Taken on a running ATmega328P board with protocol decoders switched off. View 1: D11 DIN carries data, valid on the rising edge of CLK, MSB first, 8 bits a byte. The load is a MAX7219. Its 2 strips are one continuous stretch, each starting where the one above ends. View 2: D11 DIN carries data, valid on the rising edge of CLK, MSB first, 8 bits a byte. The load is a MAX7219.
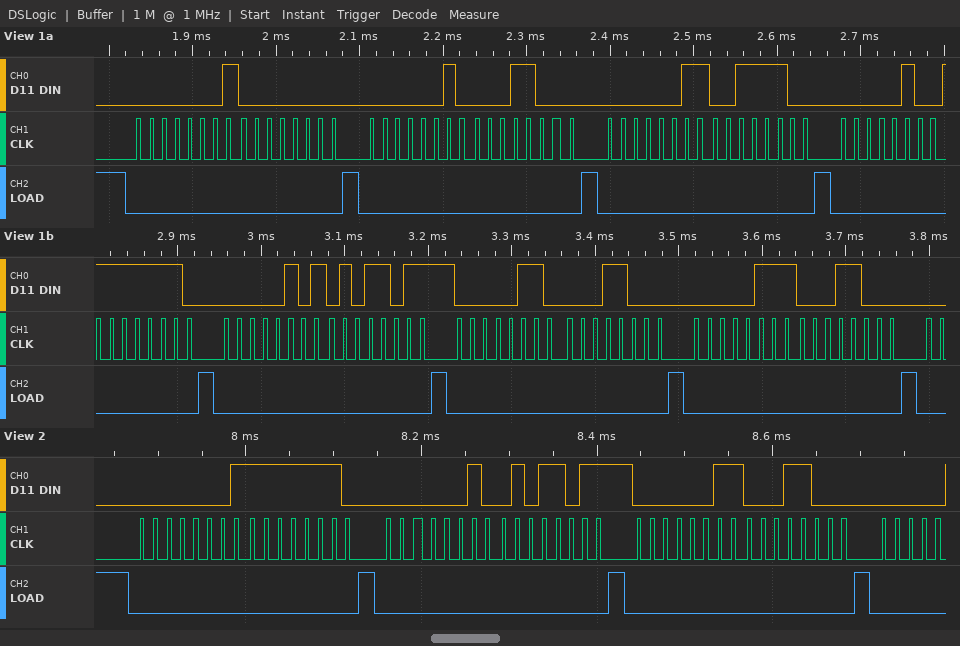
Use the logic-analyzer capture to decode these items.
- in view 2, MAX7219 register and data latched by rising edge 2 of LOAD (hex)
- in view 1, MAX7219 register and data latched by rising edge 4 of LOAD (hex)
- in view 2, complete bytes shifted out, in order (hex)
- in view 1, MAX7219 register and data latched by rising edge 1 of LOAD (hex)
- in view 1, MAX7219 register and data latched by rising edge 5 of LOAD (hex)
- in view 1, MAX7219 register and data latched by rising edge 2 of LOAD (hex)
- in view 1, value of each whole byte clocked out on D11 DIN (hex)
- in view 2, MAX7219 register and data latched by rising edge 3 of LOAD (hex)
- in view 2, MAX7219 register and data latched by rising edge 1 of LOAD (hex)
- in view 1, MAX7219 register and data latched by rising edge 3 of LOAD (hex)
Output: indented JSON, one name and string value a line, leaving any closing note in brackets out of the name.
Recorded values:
{
  "in view 2, MAX7219 register and data latched by rising edge 2 of LOAD": "register 0x2, data 0x5B",
  "in view 1, MAX7219 register and data latched by rising edge 4 of LOAD": "register 0x4, data 0xFE",
  "in view 2, complete bytes shifted out, in order": "01 FE 02 5B 03 18",
  "in view 1, MAX7219 register and data latched by rising edge 1 of LOAD": "register 0x1, data 0x00",
  "in view 1, MAX7219 register and data latched by rising edge 5 of LOAD": "register 0x5, data 0x5B",
  "in view 1, MAX7219 register and data latched by rising edge 2 of LOAD": "register 0x2, data 0x18",
  "in view 1, value of each whole byte clocked out on D11 DIN": "01 00 02 18 03 3C 04 FE 05 5B 06 18 07 18",
  "in view 2, MAX7219 register and data latched by rising edge 3 of LOAD": "register 0x3, data 0x18",
  "in view 2, MAX7219 register and data latched by rising edge 1 of LOAD": "register 0x1, data 0xFE",
  "in view 1, MAX7219 register and data latched by rising edge 3 of LOAD": "register 0x3, data 0x3C"
}
